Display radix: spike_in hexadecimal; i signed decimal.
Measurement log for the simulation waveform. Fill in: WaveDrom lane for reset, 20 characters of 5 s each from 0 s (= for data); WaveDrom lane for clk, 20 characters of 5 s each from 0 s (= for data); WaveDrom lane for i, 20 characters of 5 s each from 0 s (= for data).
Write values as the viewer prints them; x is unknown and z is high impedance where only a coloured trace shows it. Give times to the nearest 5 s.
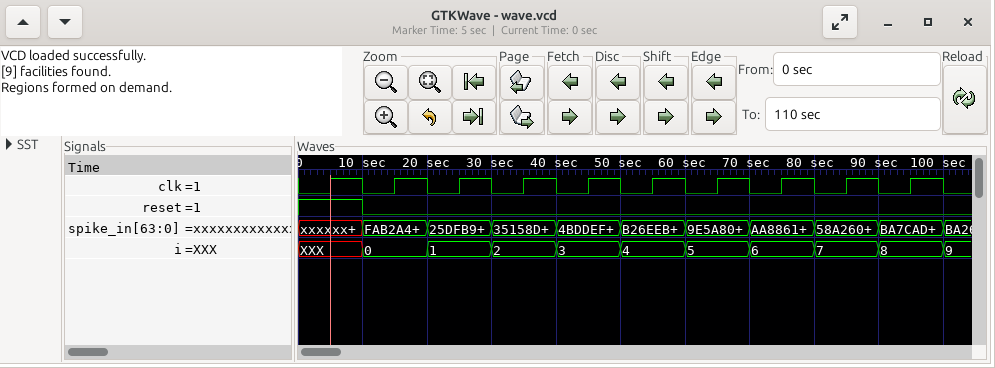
{name: 'reset', wave: '1.0.................'}
{name: 'clk', wave: '01010101010101010101'}
{name: 'i', wave: 'x.=.=.=.=.=.=.=.=.=.', data: '0 1 2 3 4 5 6 7 8'}
